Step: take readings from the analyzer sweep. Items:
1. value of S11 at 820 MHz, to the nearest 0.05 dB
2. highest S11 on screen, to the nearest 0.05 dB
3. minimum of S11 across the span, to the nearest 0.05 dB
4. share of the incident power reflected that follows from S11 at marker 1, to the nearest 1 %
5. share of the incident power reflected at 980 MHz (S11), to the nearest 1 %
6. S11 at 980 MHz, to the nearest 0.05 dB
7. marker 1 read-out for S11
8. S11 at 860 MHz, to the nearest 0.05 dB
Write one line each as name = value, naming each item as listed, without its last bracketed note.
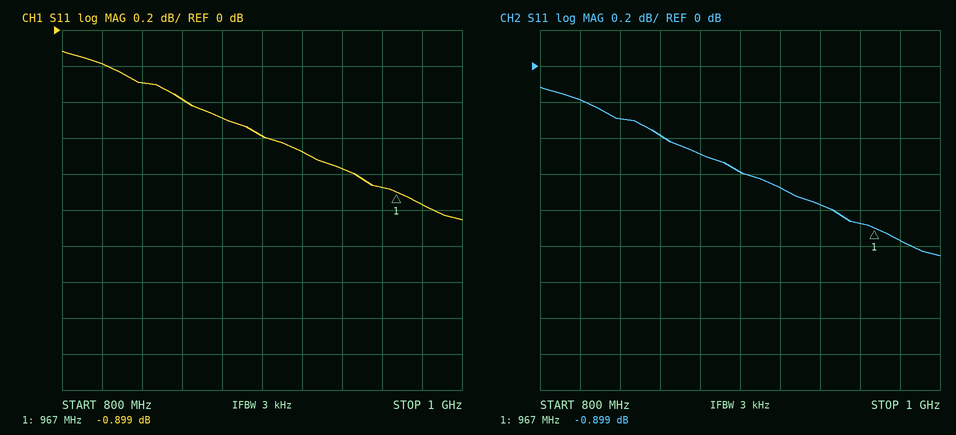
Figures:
value of S11 at 820 MHz, to the nearest 0.05 dB = -0.20 dB
highest S11 on screen, to the nearest 0.05 dB = -0.10 dB
minimum of S11 across the span, to the nearest 0.05 dB = -1.05 dB
share of the incident power reflected that follows from S11 at marker 1, to the nearest 1 % = 81 %
share of the incident power reflected at 980 MHz (S11), to the nearest 1 % = 80 %
S11 at 980 MHz, to the nearest 0.05 dB = -0.95 dB
marker 1 read-out for S11 = -0.899 dB
S11 at 860 MHz, to the nearest 0.05 dB = -0.40 dB
